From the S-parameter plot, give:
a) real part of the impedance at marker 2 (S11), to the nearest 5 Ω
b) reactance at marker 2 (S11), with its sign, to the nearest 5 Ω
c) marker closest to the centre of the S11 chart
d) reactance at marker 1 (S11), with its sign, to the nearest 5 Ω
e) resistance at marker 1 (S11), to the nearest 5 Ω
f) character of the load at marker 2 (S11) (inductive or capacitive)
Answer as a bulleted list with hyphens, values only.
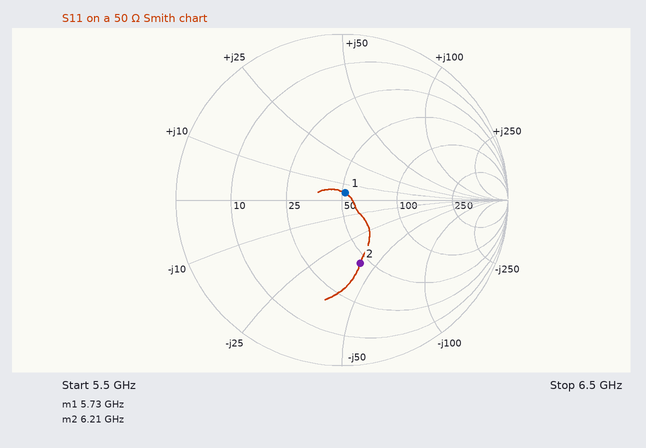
- 45 Ω
- -40 Ω
- marker 1
- +5 Ω
- 50 Ω
- capacitive
